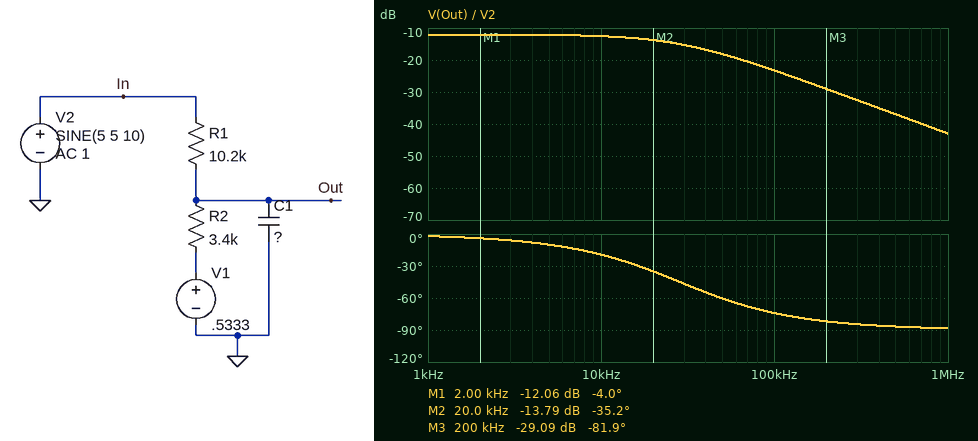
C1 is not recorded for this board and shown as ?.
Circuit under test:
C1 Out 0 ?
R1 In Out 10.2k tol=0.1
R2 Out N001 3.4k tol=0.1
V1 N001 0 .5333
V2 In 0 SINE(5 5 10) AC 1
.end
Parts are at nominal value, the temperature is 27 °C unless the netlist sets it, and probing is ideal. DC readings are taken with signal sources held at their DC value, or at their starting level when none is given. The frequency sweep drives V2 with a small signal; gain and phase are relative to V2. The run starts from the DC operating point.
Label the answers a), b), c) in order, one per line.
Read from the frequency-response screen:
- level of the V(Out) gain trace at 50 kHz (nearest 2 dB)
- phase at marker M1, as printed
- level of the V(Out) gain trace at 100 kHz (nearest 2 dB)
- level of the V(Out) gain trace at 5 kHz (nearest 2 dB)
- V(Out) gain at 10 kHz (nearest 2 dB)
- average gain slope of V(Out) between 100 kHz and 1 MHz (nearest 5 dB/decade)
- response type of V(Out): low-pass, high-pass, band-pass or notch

a) -18 dB
b) -4.0 deg
c) -24 dB
d) -12 dB
e) -12 dB
f) -20 dB/decade
g) low-pass
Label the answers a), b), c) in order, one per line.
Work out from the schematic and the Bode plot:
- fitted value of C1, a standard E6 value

a) 2.2 nF
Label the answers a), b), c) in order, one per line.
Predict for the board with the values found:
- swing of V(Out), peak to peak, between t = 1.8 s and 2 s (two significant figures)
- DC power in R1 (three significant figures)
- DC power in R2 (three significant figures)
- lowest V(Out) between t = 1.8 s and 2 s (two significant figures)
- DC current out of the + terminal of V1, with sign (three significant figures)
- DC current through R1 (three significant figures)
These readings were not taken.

a) 2.5 V
b) 1.10 mW
c) 367 µW
d) 400 mV
e) -328 µA
f) 328 µA
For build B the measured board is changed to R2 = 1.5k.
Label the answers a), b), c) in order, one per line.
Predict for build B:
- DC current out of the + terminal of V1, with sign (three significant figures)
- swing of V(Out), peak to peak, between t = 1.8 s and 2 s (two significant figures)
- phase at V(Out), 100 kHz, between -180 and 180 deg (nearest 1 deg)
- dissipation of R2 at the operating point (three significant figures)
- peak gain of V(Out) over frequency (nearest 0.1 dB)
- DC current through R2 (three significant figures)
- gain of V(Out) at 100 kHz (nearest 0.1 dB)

a) -382 µA
b) 1.3 V
c) -61 deg
d) 219 µW
e) -17.8 dB
f) 382 µA
g) -24.1 dB
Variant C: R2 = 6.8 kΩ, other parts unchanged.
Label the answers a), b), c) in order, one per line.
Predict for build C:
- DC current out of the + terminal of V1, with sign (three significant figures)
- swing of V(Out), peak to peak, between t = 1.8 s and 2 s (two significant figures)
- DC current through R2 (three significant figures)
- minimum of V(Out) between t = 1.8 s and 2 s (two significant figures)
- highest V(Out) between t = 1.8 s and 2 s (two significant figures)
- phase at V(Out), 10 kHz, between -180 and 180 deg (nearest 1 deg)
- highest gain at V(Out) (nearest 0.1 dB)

a) -263 µA
b) 4.0 V
c) 263 µA
d) 320 mV
e) 4.3 V
f) -29 deg
g) -8.0 dB
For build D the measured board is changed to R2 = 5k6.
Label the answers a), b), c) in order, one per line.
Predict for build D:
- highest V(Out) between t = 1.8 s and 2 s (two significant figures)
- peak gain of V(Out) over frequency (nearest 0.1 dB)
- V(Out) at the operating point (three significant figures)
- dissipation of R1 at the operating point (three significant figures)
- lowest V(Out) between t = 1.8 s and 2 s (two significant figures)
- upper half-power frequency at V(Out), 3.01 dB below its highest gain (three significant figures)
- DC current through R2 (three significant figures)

a) 3.9 V
b) -9.0 dB
c) 2.12 V
d) 815 µW
e) 340 mV
f) 20.0 kHz
g) 283 µA
